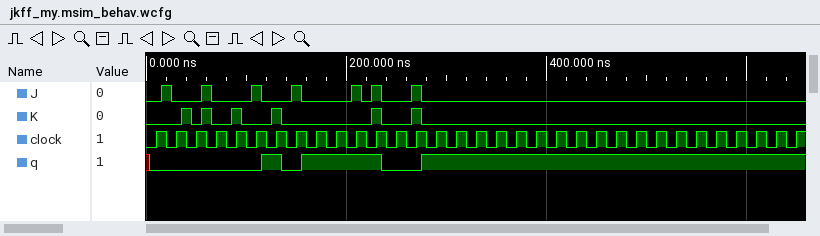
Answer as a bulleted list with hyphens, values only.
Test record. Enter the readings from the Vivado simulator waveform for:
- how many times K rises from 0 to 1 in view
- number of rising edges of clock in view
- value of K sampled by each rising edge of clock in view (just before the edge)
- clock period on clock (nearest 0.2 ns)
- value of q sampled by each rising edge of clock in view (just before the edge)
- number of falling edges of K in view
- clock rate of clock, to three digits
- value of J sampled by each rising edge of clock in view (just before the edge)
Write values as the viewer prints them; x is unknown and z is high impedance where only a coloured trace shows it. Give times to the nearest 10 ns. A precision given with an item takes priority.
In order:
- 6
- 33
- 0 0 0 0 1 0 1 0 0 0 0 1 0 1 0 0 0 0 0 0 0 0 0 0 0 0 0 0 0 0 0 0 0
- 20 ns
- 0 0 0 0 0 0 1 0 1 1 1 1 0 0 1 1 1 1 1 1 1 1 1 1 1 1 1 1 1 1 1 1 1
- 6
- 50.0 MHz
- 0 0 0 0 0 1 0 1 0 0 1 1 0 1 0 0 0 0 0 0 0 0 0 0 0 0 0 0 0 0 0 0 0
